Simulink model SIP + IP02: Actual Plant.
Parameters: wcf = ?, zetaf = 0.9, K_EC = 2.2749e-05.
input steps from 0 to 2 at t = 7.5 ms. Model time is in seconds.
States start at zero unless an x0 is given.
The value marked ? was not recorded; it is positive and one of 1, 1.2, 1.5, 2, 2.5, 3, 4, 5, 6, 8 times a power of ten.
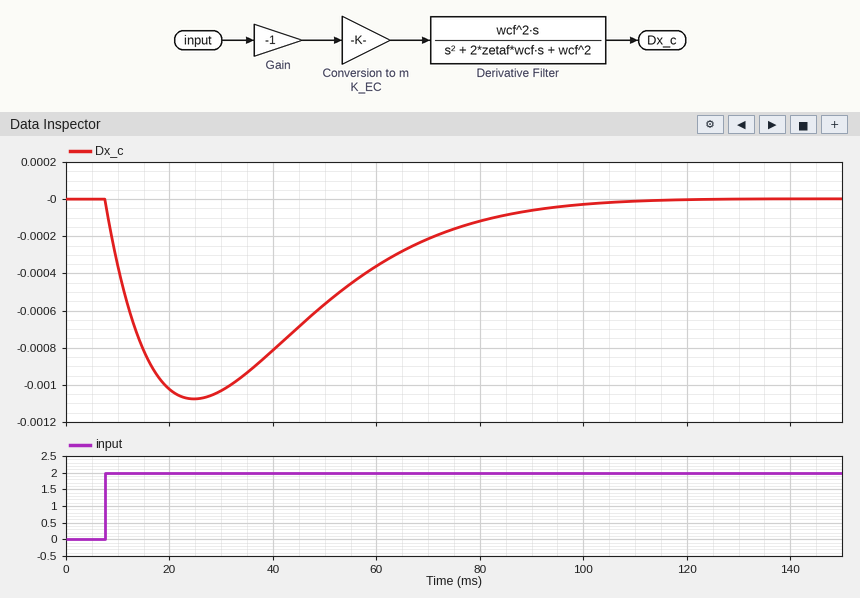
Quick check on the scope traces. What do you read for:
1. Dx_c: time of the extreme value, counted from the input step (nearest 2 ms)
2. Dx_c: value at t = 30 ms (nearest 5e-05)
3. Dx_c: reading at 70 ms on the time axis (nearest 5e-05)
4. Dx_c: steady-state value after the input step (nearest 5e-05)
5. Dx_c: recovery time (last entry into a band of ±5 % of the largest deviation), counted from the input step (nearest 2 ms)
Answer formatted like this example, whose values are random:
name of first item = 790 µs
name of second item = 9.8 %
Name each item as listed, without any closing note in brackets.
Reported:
Dx_c: time of the extreme value, counted from the input step = 18 ms
Dx_c: value at t = 30 ms = -0.00105
Dx_c: reading at 70 ms on the time axis = -0.00020
Dx_c: steady-state value after the input step = 0.00000
Dx_c: recovery time (last entry into a band of ±5 % of the largest deviation), counted from the input step = 84 ms
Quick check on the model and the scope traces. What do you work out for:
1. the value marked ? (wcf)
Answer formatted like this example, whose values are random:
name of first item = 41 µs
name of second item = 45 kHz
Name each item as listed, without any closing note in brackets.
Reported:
the value marked ? = 60
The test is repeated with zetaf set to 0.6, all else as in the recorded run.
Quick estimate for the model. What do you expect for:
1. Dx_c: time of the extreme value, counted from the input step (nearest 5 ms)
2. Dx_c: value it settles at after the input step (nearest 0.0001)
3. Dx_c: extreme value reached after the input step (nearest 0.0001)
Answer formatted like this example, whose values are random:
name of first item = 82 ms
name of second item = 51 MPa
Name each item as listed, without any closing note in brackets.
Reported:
Dx_c: time of the extreme value, counted from the input step = 20 ms
Dx_c: value it settles at after the input step = 0.0000
Dx_c: extreme value reached after the input step = -0.0014
